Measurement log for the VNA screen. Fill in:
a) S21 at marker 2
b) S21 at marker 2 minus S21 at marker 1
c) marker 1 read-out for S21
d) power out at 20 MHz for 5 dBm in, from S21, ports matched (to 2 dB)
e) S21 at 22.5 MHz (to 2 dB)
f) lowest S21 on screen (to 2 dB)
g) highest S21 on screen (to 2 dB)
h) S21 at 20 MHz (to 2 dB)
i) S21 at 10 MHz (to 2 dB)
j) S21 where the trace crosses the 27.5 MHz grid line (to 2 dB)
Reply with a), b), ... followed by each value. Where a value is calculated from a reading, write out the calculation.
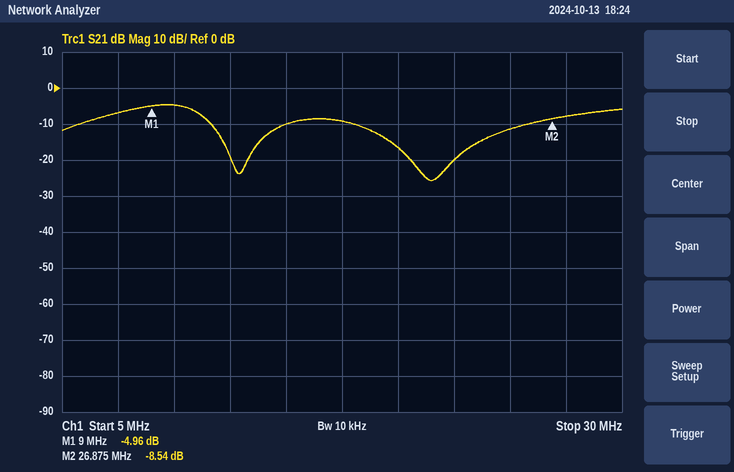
a) -8.54 dB
b) -8.54 − (-4.96) = -3.58 dB
c) -4.96 dB
d) 5 dBm + (-16 dB) = -12 dBm
e) -20 dB
f) -26 dB
g) -4 dB
h) -16 dB
i) -4 dB
j) -8 dB
